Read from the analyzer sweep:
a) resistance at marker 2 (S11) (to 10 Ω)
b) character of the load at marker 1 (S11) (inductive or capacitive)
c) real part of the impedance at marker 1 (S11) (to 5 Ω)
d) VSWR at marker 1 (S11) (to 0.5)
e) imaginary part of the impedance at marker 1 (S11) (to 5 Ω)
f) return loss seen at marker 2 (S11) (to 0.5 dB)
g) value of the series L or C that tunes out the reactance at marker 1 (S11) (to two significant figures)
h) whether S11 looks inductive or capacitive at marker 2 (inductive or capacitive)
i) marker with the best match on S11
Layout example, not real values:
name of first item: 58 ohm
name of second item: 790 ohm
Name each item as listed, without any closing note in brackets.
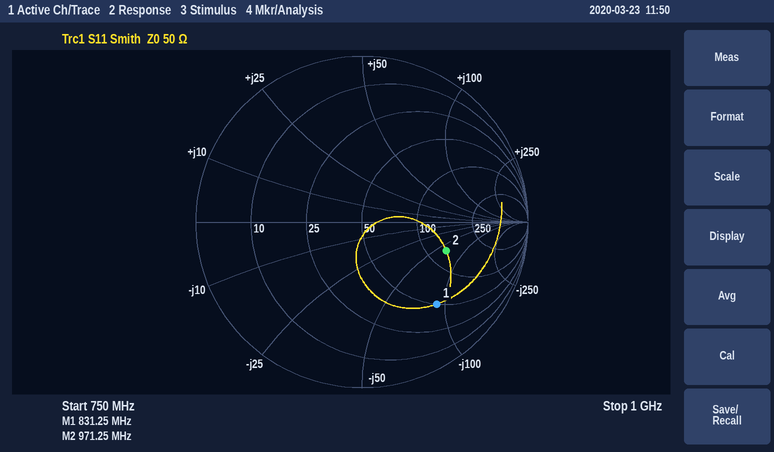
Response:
resistance at marker 2 (S11): 130 Ω
character of the load at marker 1 (S11): capacitive
real part of the impedance at marker 1 (S11): 50 Ω
VSWR at marker 1 (S11): 5.0
imaginary part of the impedance at marker 1 (S11): -90 Ω
return loss seen at marker 2 (S11): 5.5 dB
value of the series L or C that tunes out the reactance at marker 1 (S11): 17 nH
whether S11 looks inductive or capacitive at marker 2: capacitive
marker with the best match on S11: marker 2
